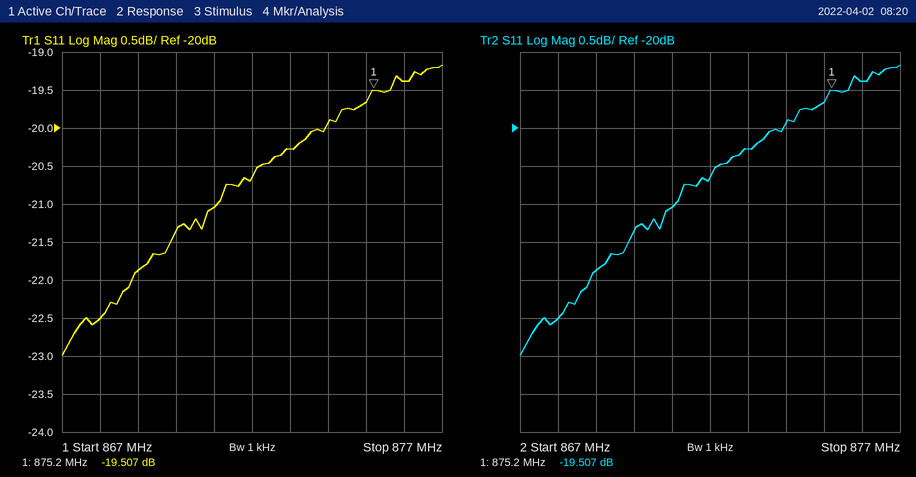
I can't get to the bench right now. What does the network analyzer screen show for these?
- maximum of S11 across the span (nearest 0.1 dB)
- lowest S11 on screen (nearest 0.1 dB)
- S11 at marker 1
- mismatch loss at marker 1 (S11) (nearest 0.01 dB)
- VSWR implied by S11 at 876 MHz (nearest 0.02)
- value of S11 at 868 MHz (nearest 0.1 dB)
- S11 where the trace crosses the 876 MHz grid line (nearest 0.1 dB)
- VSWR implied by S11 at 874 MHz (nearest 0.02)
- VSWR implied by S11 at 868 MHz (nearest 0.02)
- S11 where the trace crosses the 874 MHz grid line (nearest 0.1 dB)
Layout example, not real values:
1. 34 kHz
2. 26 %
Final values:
1. -19.2 dB
2. -23.0 dB
3. -19.507 dB
4. 0.05 dB
5. 1.24
6. -22.5 dB
7. -19.4 dB
8. 1.22
9. 1.16
10. -19.9 dB
